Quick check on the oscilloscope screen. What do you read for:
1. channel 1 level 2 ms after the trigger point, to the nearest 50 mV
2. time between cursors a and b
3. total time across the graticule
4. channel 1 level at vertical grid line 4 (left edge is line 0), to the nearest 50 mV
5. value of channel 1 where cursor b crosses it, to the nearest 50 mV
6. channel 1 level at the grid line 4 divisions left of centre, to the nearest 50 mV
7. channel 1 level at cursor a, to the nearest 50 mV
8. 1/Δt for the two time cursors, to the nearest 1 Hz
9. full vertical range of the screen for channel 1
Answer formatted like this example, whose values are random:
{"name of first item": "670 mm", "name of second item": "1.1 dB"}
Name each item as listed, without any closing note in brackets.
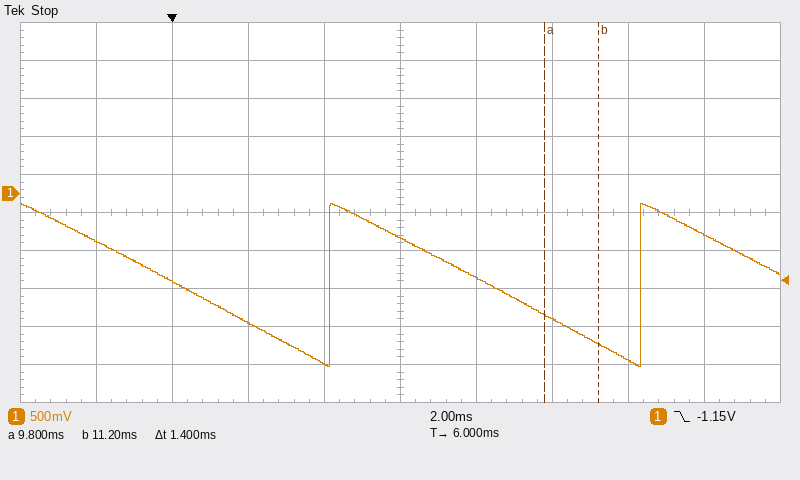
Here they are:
{"channel 1 level 2 ms after the trigger point, to the nearest 50 mV": "-1.70 V", "time between cursors a and b": "1.4 ms", "total time across the graticule": "20 ms", "channel 1 level at vertical grid line 4 (left edge is line 0), to the nearest 50 mV": "-2.25 V", "value of channel 1 where cursor b crosses it, to the nearest 50 mV": "-2.00 V", "channel 1 level at the grid line 4 divisions left of centre, to the nearest 50 mV": "-650 mV", "channel 1 level at cursor a, to the nearest 50 mV": "-1.60 V", "1/Δt for the two time cursors, to the nearest 1 Hz": "714 Hz", "full vertical range of the screen for channel 1": "5 V"}
